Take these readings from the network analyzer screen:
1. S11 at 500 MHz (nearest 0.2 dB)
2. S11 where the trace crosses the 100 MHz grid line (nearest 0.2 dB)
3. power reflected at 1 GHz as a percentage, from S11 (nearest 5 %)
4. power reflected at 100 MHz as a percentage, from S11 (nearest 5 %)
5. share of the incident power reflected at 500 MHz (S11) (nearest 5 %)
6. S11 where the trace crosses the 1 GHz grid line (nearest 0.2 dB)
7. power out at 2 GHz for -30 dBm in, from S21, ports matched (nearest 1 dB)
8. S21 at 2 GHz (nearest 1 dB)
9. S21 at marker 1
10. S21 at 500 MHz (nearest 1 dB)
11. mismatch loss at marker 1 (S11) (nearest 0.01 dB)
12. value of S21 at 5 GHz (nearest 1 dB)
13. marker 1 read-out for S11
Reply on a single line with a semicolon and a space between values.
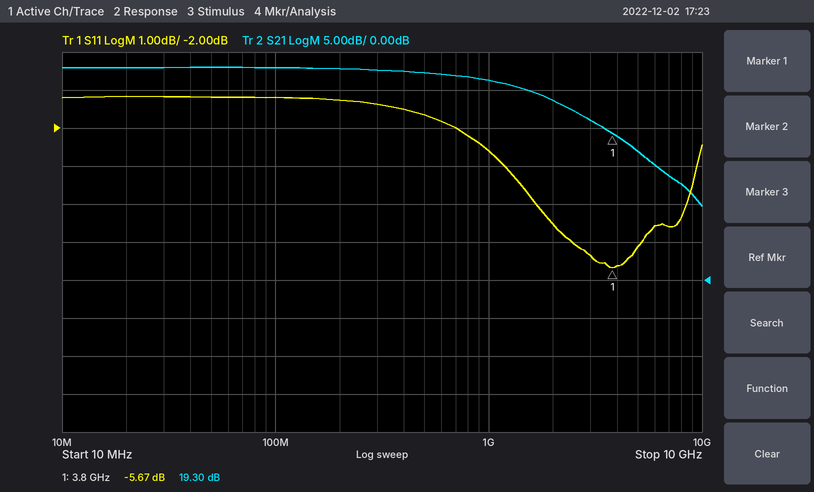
-1.6 dB; -1.2 dB; 55 %; 75 %; 70 %; -2.6 dB; -6 dBm; 24 dB; 19.30 dB; 27 dB; 1.37 dB; 17 dB; -5.67 dB
